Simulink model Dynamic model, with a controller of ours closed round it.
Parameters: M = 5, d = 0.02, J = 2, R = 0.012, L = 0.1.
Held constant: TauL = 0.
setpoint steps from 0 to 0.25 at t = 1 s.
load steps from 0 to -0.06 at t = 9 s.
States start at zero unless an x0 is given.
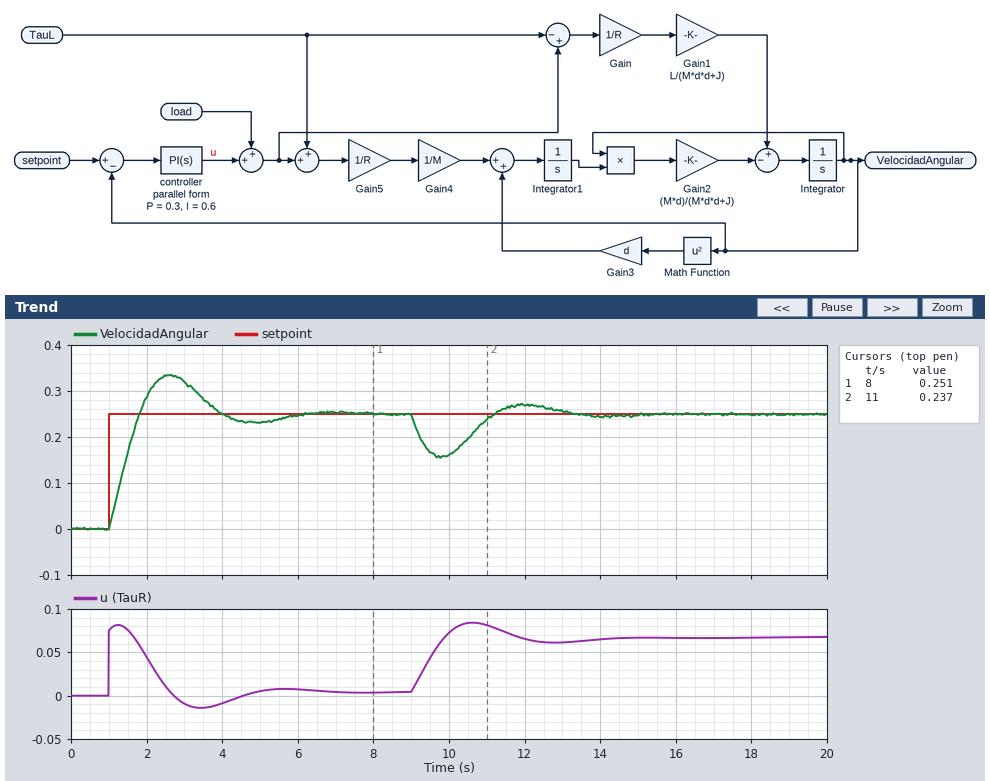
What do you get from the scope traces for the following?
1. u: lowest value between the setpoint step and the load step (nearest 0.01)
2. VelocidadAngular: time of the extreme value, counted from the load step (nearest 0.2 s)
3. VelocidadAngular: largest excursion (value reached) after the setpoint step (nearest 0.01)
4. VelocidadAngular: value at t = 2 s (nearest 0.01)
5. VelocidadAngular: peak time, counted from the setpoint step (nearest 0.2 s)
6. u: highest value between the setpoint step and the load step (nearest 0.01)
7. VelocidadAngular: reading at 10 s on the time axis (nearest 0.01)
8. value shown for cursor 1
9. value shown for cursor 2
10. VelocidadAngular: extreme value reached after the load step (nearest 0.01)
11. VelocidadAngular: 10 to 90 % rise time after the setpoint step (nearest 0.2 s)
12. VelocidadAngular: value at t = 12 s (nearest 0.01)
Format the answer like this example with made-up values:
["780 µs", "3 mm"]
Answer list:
["-0.01", "0.8 s", "0.33", "0.29", "1.6 s", "0.08", "0.16", "0.251", "0.237", "0.16", "0.6 s", "0.27"]
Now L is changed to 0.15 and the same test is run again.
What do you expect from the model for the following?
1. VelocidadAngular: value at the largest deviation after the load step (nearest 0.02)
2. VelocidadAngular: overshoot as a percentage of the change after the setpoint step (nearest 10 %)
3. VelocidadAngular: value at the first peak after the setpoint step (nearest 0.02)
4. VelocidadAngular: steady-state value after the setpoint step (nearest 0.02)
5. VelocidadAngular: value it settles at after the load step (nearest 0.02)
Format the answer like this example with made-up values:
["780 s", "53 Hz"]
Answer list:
["0.14", "30 %", "0.32", "0.24", "0.24"]
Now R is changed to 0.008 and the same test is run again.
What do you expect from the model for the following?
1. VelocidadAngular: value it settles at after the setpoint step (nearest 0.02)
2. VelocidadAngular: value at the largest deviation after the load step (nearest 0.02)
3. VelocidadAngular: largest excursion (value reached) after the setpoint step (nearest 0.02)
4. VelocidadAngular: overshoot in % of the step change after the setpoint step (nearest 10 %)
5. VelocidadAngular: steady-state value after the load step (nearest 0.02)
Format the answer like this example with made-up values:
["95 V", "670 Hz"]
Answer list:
["0.24", "0.14", "0.32", "40 %", "0.24"]
